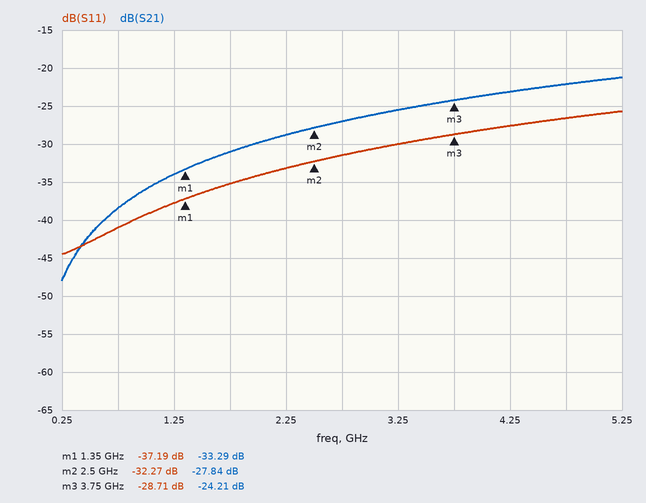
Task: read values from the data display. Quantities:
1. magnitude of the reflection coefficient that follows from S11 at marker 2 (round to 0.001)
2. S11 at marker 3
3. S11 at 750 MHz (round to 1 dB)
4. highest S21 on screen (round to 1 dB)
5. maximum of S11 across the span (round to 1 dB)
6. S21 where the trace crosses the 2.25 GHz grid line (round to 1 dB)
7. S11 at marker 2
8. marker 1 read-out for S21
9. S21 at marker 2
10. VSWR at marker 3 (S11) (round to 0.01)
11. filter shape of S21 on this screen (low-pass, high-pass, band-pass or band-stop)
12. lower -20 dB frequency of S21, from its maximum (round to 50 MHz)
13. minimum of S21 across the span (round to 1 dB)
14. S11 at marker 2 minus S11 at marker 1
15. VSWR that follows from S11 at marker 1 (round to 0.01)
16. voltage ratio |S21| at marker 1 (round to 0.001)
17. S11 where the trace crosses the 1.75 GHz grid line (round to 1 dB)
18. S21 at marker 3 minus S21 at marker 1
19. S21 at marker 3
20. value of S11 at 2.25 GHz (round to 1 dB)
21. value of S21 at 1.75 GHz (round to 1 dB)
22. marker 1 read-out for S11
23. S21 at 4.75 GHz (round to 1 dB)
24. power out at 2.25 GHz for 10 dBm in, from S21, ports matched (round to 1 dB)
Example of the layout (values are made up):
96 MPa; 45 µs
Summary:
0.024; -28.71 dB; -41 dB; -21 dB; -26 dB; -29 dB; -32.27 dB; -33.29 dB; -27.84 dB; 1.08; high-pass; 550 MHz; -48 dB; 4.92 dB; 1.03; 0.022; -35 dB; 9.08 dB; -24.21 dB; -33 dB; -31 dB; -37.19 dB; -22 dB; -19 dBm
